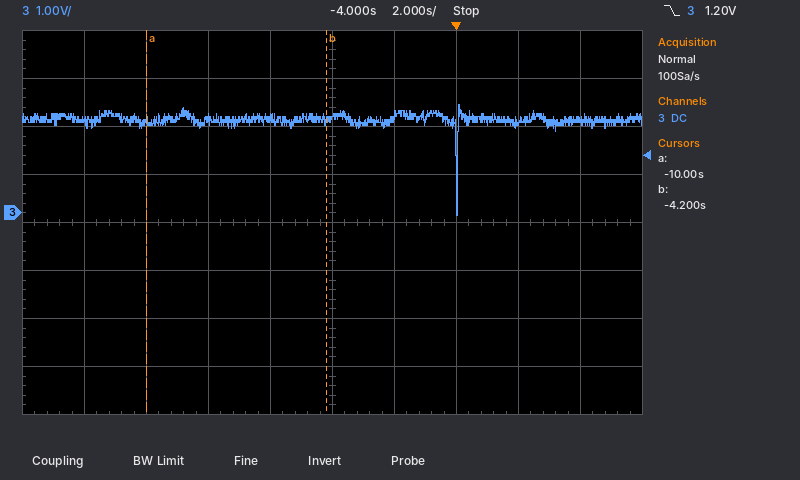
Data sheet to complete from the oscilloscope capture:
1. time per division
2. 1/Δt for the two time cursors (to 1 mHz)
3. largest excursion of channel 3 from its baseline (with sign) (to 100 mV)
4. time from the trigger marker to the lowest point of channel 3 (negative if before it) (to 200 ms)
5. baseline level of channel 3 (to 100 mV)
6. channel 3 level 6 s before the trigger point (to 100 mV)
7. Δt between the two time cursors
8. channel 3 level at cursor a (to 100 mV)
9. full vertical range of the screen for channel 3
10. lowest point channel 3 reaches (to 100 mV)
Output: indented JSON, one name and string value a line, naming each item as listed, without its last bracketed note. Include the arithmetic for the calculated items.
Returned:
{
  "time per division": "2 s",
  "1/Δt for the two time cursors": "1 / 5.8 s ≈ 172 mHz",
  "largest excursion of channel 3 from its baseline (with sign)": "-100 mV − (1.9 V) = -2.0 V",
  "time from the trigger marker to the lowest point of channel 3 (negative if before it)": "0.0 s",
  "baseline level of channel 3": "1.9 V",
  "channel 3 level 6 s before the trigger point": "2.0 V",
  "Δt between the two time cursors": "-4.2 s − (-10 s) = 5.8 s",
  "channel 3 level at cursor a": "1.9 V",
  "full vertical range of the screen for channel 3": "8 V",
  "lowest point channel 3 reaches": "-100 mV"
}
